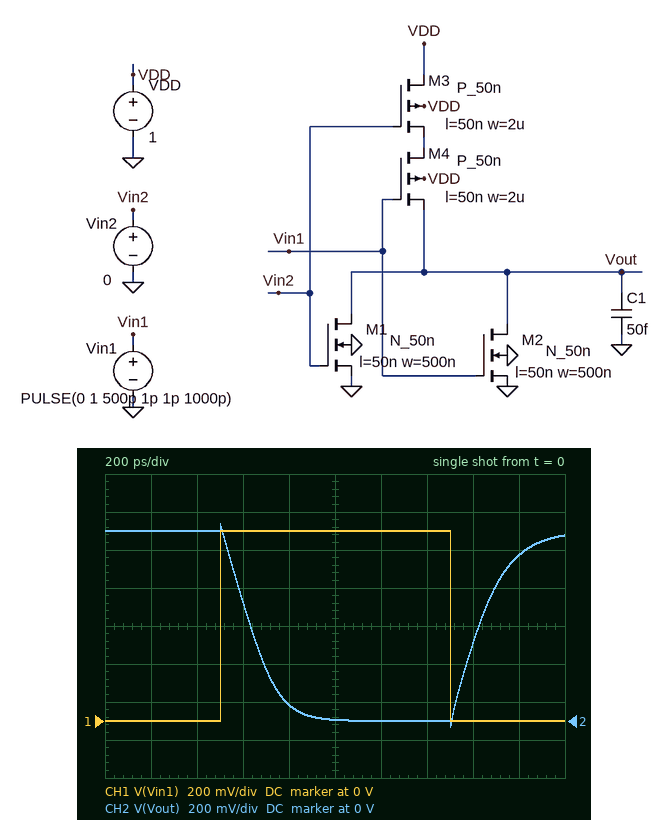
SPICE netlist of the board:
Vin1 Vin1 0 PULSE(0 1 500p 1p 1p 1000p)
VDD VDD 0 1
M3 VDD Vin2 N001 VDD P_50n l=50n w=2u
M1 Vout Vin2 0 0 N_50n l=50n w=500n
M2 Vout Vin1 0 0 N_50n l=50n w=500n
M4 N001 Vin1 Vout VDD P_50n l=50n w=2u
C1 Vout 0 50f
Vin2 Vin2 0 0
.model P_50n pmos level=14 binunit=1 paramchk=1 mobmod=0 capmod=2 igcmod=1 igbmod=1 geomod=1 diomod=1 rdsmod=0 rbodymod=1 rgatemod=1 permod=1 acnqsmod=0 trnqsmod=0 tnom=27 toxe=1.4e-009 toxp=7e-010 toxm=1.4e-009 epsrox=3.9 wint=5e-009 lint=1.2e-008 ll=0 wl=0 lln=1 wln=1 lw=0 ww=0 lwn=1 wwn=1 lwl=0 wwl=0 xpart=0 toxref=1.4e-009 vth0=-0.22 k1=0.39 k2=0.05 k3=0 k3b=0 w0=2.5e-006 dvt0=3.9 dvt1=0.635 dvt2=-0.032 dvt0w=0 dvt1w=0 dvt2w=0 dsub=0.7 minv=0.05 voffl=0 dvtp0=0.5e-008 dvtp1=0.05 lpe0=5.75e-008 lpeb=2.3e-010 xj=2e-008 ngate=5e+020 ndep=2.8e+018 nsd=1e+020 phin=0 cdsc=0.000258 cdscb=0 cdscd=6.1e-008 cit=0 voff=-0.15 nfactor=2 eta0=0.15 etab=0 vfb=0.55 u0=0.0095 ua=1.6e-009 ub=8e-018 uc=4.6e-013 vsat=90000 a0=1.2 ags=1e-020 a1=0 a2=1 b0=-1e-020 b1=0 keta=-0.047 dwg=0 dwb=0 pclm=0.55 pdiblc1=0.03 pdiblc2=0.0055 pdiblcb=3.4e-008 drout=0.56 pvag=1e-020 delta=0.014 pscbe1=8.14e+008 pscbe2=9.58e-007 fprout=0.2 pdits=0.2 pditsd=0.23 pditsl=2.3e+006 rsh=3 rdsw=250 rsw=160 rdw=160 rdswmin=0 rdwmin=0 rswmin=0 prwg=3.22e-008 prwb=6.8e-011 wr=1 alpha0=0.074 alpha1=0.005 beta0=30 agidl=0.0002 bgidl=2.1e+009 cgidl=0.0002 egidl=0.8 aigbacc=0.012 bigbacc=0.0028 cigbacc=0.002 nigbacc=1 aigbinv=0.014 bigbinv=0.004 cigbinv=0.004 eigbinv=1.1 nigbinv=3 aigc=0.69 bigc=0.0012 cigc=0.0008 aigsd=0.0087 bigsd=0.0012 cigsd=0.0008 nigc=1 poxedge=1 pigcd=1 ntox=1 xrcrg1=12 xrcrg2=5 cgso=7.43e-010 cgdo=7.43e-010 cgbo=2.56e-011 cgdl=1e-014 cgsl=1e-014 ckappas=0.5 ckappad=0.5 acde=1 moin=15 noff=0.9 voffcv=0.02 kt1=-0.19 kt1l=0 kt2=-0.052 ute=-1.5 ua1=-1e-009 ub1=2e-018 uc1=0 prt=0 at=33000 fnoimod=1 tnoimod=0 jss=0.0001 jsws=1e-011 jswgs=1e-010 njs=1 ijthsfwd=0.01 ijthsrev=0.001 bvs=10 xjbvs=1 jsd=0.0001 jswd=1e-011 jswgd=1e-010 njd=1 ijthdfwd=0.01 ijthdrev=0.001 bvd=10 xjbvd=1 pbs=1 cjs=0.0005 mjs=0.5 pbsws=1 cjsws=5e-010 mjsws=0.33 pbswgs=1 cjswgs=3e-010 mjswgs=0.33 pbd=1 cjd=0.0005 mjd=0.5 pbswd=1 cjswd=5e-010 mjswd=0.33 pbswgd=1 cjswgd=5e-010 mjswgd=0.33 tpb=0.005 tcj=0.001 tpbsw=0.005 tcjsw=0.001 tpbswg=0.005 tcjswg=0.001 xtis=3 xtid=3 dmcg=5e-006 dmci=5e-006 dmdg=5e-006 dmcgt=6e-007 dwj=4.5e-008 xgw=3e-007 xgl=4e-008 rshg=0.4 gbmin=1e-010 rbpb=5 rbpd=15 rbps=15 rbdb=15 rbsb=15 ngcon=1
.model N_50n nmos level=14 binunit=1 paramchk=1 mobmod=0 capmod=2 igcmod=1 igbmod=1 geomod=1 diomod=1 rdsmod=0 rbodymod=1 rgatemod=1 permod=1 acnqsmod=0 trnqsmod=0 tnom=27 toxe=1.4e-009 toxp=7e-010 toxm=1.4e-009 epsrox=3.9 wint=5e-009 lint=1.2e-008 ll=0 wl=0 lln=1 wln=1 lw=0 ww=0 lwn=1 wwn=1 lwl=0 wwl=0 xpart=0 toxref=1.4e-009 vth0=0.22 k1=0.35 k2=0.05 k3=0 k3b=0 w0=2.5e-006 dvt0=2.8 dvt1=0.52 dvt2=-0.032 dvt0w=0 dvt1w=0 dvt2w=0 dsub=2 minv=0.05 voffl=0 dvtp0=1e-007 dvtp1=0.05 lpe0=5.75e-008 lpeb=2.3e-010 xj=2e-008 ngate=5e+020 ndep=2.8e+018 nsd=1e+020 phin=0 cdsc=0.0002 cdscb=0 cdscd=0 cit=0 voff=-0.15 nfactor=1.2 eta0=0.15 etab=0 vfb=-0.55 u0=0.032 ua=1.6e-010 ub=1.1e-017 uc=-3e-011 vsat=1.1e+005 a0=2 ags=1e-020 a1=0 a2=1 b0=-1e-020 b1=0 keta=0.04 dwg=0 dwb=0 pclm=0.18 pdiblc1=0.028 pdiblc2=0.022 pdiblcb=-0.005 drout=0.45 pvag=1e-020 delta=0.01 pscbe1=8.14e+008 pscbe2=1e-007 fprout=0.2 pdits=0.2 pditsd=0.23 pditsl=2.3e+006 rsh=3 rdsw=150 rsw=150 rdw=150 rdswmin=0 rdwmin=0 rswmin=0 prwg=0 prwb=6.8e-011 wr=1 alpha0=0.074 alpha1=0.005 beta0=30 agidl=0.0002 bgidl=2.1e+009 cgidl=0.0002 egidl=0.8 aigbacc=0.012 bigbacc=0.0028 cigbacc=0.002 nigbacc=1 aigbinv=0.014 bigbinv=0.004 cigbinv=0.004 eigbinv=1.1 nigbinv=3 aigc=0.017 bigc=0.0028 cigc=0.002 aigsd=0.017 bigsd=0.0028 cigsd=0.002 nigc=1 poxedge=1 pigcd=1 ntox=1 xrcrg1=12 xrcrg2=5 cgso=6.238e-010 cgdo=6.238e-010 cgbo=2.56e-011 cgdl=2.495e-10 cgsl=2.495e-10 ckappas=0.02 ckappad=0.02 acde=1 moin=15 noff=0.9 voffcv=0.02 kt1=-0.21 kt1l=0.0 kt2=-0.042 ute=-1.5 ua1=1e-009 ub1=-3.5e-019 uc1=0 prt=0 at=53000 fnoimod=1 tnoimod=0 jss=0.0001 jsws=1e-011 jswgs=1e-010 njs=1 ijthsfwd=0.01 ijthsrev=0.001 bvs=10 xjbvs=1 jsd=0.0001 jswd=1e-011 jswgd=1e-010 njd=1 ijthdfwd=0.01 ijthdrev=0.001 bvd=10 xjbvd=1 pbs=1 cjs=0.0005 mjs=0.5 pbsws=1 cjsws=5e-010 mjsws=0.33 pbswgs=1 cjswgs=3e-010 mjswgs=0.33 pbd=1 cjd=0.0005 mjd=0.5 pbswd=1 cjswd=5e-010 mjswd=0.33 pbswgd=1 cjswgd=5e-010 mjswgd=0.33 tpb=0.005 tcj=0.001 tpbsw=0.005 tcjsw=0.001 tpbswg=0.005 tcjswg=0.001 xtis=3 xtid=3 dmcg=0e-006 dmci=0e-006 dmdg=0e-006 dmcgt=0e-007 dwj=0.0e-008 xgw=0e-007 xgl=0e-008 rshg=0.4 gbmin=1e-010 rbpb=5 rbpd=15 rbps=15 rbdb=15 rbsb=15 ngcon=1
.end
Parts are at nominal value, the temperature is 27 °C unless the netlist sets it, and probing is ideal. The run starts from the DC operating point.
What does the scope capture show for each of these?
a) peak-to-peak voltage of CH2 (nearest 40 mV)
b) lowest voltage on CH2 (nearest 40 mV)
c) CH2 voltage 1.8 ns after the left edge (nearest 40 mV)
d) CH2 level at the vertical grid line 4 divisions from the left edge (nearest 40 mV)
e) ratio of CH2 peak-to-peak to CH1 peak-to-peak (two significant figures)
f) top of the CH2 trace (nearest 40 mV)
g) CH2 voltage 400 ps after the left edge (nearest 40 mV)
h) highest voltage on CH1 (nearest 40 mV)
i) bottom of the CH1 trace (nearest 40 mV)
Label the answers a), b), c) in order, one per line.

a) 1.08 V
b) -40 mV
c) 880 mV
d) 80 mV
e) 1.1
f) 1.04 V
g) 1.00 V
h) 1.00 V
i) 0 V
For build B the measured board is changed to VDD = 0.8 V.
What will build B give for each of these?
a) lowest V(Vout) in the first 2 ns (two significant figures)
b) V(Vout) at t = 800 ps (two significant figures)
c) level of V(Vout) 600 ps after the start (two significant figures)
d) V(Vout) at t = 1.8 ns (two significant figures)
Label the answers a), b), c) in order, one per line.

a) -34 mV
b) 48 mV
c) 450 mV
d) 630 mV
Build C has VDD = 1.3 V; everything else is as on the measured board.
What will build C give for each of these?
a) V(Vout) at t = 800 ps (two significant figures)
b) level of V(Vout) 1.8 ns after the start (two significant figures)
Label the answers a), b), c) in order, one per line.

a) 200 mV
b) 1.2 V
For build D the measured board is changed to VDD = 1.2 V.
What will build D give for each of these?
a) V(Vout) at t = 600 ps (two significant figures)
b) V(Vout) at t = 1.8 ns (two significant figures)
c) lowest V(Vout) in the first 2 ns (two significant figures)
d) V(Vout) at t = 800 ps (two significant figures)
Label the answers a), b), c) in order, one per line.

a) 810 mV
b) 1.1 V
c) -31 mV
d) 150 mV
